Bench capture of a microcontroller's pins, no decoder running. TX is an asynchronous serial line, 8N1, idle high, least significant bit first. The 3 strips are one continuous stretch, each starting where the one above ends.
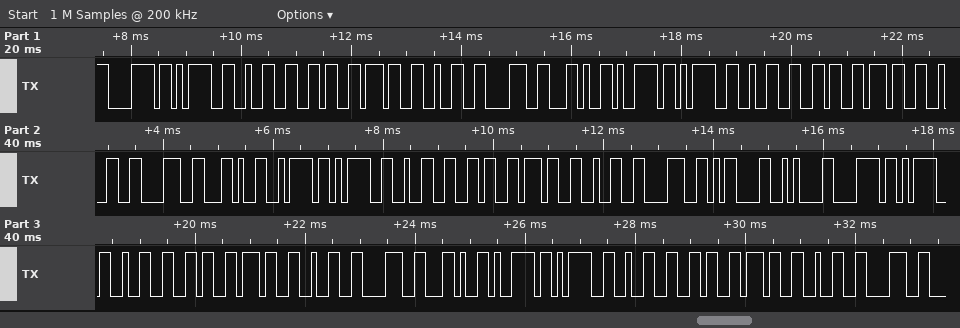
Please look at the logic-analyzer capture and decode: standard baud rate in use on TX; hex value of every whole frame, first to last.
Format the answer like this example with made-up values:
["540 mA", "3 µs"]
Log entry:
["9600 baud", "78 3D 32 36 37 32 38 2C 79 3D 32 36 37 32 38 2C 7A 3D 32 36 37 32 38 0D 0A 78 3D 32 36 37 32 38 2C 79 3D 32 36 37 32 38"]
